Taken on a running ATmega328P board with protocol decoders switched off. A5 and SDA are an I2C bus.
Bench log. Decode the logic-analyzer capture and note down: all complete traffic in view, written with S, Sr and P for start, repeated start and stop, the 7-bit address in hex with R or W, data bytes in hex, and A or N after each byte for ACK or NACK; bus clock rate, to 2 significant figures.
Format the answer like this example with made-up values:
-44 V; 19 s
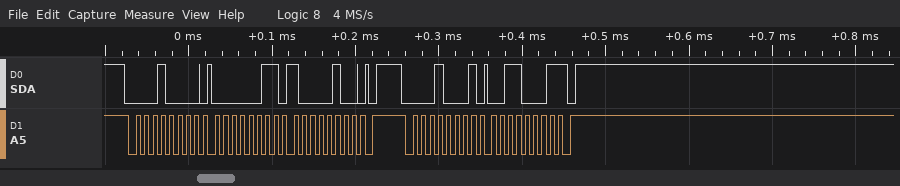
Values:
S 08W A 03 A 84 A P S 08R A 31 N P; 100 kHz
